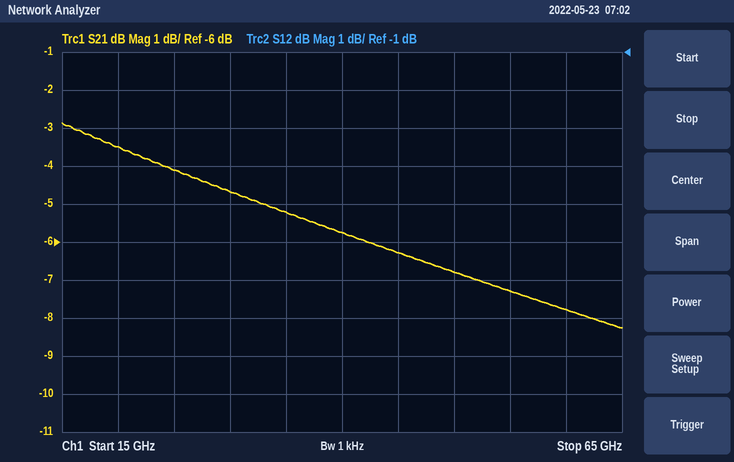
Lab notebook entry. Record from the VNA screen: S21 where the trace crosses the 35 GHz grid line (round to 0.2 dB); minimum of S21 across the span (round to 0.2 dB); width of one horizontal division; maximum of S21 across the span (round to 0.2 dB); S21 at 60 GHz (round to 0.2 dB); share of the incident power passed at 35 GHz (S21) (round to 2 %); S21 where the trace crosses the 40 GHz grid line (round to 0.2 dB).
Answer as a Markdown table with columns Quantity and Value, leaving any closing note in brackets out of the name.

| Quantity | Value |
|---|---|
| S21 where the trace crosses the 35 GHz grid line | -5.2 dB |
| minimum of S21 across the span | -8.2 dB |
| width of one horizontal division | 5 GHz |
| maximum of S21 across the span | -2.8 dB |
| S21 at 60 GHz | -7.8 dB |
| share of the incident power passed at 35 GHz (S21) | 30 % |
| S21 where the trace crosses the 40 GHz grid line | -5.8 dB |
